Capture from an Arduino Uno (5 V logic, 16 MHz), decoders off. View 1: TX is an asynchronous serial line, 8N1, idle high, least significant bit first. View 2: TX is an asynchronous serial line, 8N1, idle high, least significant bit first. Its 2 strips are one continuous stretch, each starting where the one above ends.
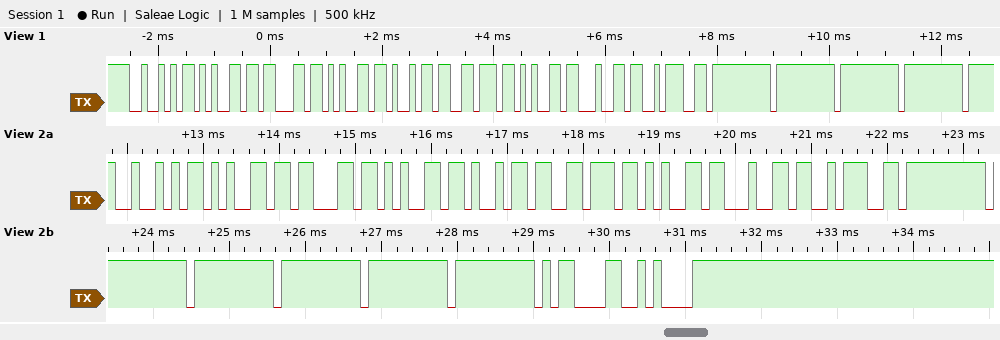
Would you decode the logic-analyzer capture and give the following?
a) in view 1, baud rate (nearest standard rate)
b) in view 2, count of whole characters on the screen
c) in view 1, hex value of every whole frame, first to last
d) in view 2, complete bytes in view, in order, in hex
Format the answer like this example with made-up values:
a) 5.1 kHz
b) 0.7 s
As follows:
a) 9600 baud
b) 17
c) 52 65 63 65 69 76 65 64 3A FF FF FF FF
d) 52 65 63 65 69 76 65 64 3A FF FF FF FF FF FF 0D 0A
